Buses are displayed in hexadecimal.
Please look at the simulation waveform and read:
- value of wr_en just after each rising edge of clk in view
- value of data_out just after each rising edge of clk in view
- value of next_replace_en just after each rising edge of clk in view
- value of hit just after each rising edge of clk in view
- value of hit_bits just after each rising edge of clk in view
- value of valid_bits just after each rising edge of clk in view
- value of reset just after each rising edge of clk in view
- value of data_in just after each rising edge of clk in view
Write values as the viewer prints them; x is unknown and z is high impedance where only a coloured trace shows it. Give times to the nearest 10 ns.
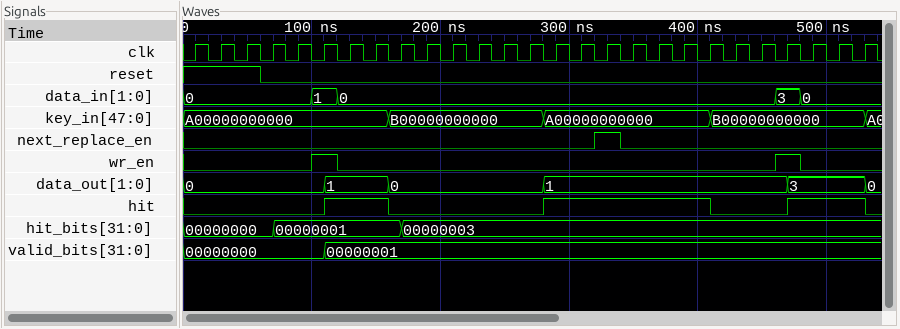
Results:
0 0 0 0 0 1 0 0 0 0 0 0 0 0 0 0 0 0 0 0 0 0 0 1 0 0 0
0, 0, 0, 0, 0, 1, 1, 1, 0, 0, 0, 0, 0, 0, 1, 1, 1, 1, 1, 1, 1, 1, 1, 3, 3, 3, 0
0 0 0 0 0 0 0 0 0 0 0 0 0 0 0 0 1 0 0 0 0 0 0 0 0 0 0
0 0 0 0 0 1 1 1 0 0 0 0 0 0 1 1 1 1 1 1 0 0 0 1 1 1 0
00000000, 00000000, 00000000, 00000001, 00000001, 00000001, 00000001, 00000001, 00000003, 00000003, 00000003, 00000003, 00000003, 00000003, 00000003, 00000003, 00000003, 00000003, 00000003, 00000003, 00000003, 00000003, 00000003, 00000003, 00000003, 00000003, 00000003
00000000, 00000000, 00000000, 00000000, 00000000, 00000001, 00000001, 00000001, 00000001, 00000001, 00000001, 00000001, 00000001, 00000001, 00000001, 00000001, 00000001, 00000001, 00000001, 00000001, 00000001, 00000001, 00000001, 00000001, 00000001, 00000001, 00000001
1 1 1 0 0 0 0 0 0 0 0 0 0 0 0 0 0 0 0 0 0 0 0 0 0 0 0
0, 0, 0, 0, 0, 1, 0, 0, 0, 0, 0, 0, 0, 0, 0, 0, 0, 0, 0, 0, 0, 0, 0, 3, 0, 0, 0
